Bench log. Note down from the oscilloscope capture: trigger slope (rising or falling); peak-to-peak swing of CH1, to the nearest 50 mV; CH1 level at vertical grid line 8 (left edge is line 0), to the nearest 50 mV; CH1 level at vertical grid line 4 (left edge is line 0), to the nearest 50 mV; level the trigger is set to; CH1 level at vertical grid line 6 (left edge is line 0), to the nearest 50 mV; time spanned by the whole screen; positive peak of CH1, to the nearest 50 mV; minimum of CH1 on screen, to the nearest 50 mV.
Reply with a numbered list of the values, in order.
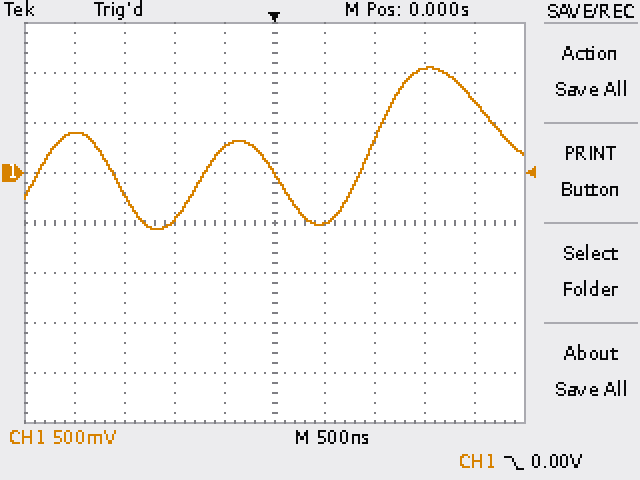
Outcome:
1. falling
2. 1.60 V
3. 1.05 V
4. 250 mV
5. 0.00 V
6. -500 mV
7. 5 µs
8. 1.05 V
9. -550 mV
